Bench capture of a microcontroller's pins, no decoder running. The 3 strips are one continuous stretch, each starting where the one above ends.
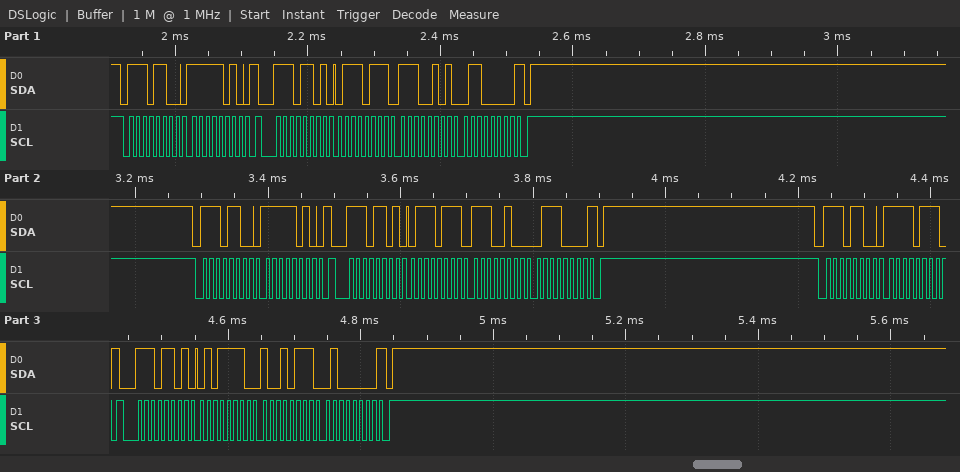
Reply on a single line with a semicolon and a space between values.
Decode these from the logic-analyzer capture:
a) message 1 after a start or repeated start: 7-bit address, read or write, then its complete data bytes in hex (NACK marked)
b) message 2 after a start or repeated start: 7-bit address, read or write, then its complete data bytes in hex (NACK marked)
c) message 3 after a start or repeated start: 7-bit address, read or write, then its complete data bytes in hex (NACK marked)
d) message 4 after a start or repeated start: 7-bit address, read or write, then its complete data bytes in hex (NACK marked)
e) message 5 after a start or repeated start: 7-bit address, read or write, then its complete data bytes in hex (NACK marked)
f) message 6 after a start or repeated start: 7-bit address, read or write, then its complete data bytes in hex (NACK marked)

0x76 write: FA; 0x76 read: 77 E5 60 NACK; 0x76 write: FA; 0x76 read: 77 E4 70 NACK; 0x76 write: F7; 0x76 read: 5E 97 40 NACK
